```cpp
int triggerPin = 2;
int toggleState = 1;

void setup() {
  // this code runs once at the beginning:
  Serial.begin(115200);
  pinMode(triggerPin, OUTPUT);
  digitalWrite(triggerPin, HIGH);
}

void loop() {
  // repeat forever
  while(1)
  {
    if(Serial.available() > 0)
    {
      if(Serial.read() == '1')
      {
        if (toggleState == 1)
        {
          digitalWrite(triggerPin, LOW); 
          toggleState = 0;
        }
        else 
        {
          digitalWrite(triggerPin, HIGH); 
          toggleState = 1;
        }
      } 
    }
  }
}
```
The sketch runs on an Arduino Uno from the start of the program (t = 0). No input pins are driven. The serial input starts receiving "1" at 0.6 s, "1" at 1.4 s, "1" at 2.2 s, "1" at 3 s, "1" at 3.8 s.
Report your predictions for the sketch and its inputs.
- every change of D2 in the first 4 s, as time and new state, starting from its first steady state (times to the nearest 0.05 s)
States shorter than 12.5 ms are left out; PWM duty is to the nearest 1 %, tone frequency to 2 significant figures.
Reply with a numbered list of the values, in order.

1. 0 s high; 0.6 s low; 1.4 s high; 2.2 s low; 3 s high; 3.8 s low
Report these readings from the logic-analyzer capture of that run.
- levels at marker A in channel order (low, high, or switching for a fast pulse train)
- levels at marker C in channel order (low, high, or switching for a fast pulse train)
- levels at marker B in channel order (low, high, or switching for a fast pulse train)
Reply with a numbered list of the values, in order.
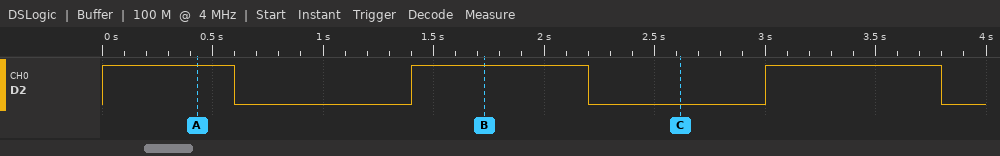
1. D2 high
2. D2 low
3. D2 high
